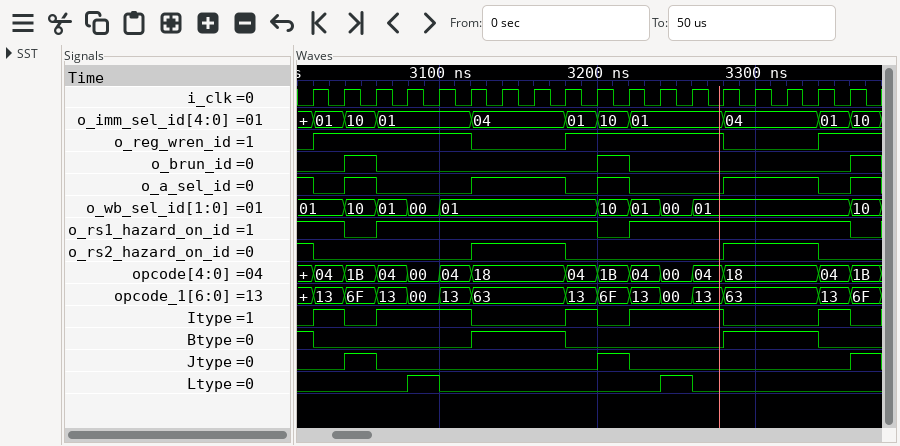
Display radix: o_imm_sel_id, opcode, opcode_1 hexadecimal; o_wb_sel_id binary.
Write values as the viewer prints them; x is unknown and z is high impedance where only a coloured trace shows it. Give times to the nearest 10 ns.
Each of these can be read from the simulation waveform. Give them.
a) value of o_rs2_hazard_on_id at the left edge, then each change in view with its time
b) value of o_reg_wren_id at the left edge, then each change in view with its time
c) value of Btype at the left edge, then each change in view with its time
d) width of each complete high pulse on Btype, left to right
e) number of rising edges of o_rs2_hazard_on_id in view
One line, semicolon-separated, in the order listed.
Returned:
1, 0 at 3020 ns, 1 at 3120 ns, 0 at 3180 ns, 1 at 3280 ns, 0 at 3340 ns; 0, 1 at 3020 ns, 0 at 3120 ns, 1 at 3180 ns, 0 at 3280 ns, 1 at 3340 ns; 1, 0 at 3020 ns, 1 at 3120 ns, 0 at 3180 ns, 1 at 3280 ns, 0 at 3340 ns; 60 ns, 60 ns; 2
